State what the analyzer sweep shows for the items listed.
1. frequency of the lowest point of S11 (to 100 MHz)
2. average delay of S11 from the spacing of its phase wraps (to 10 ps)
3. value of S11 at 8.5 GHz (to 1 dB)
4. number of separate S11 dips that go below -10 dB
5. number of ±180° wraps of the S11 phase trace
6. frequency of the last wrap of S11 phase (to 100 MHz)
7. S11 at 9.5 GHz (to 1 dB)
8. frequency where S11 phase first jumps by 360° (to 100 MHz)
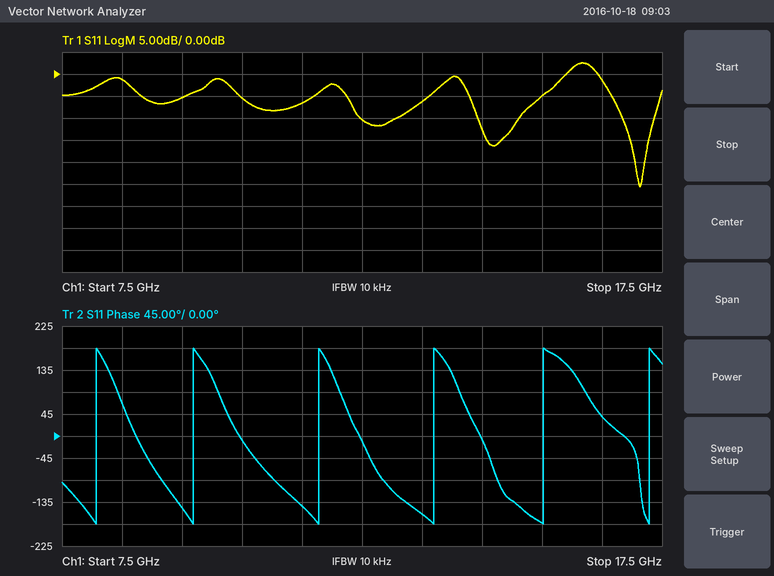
17.1 GHz
540 ps
-1 dB
3
6
17.3 GHz
-5 dB
8.1 GHz
